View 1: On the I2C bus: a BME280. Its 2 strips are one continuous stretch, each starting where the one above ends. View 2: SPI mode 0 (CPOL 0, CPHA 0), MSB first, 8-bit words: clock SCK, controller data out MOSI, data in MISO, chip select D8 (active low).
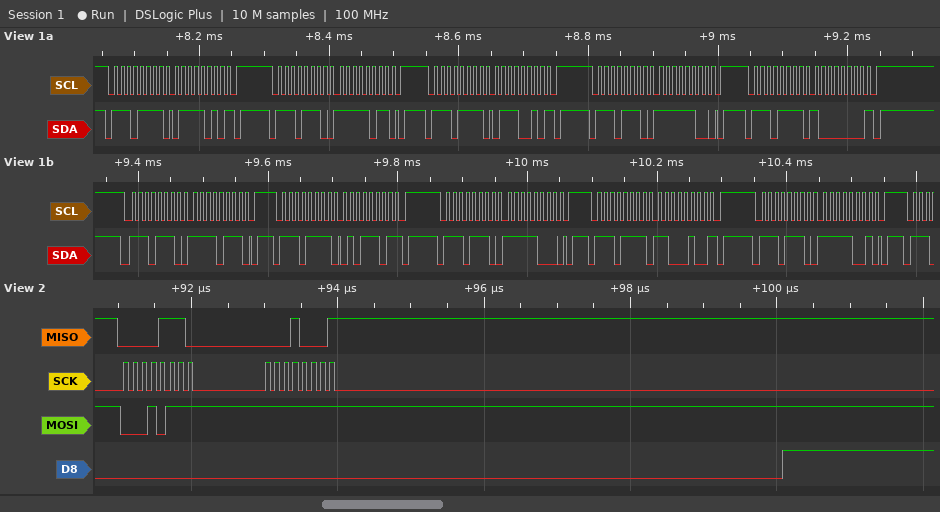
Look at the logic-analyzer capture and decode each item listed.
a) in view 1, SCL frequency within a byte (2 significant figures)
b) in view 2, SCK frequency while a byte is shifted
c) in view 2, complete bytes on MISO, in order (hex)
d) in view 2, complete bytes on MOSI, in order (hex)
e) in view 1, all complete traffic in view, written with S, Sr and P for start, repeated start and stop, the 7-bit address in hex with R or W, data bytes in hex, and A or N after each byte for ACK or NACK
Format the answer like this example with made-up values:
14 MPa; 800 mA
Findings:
100 kHz; 8 MHz; 0x0E 0x11; 0x17 0xFF; S 77R A 7A N P S 77W A FB A P S 77R A 72 N P S 77W A FC A P S 77R A 80 N P S 77W A F7 A P S 77R A 5D N P S 77W A F8 A P S 77R A C4 N P S 77W A F9 A P
